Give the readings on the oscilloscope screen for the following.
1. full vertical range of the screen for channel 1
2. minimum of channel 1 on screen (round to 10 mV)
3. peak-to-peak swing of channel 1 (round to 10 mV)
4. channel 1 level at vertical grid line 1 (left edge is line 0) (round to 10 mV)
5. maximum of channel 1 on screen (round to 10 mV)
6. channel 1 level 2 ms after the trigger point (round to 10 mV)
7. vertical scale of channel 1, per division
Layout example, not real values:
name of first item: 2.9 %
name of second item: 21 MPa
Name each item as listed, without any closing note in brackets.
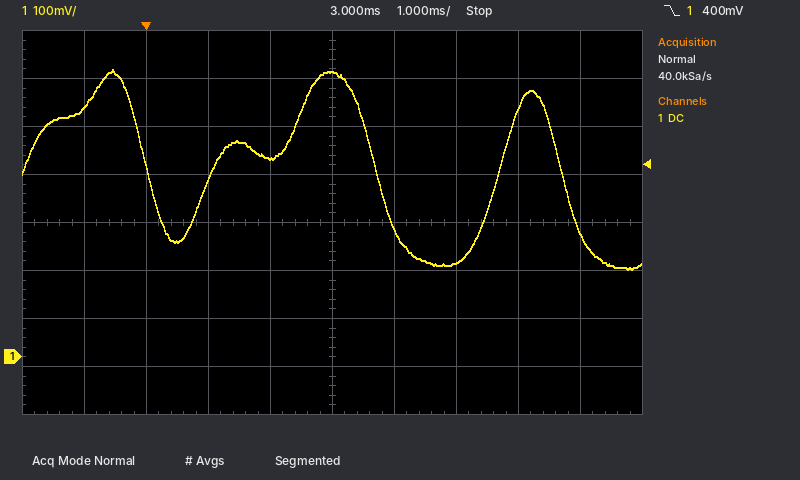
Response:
full vertical range of the screen for channel 1: 800 mV
minimum of channel 1 on screen: 180 mV
peak-to-peak swing of channel 1: 420 mV
channel 1 level at vertical grid line 1 (left edge is line 0): 520 mV
maximum of channel 1 on screen: 600 mV
channel 1 level 2 ms after the trigger point: 410 mV
vertical scale of channel 1, per division: 100 mV
